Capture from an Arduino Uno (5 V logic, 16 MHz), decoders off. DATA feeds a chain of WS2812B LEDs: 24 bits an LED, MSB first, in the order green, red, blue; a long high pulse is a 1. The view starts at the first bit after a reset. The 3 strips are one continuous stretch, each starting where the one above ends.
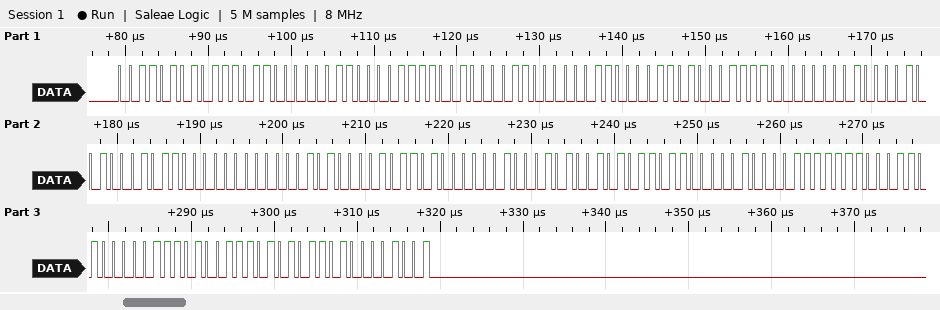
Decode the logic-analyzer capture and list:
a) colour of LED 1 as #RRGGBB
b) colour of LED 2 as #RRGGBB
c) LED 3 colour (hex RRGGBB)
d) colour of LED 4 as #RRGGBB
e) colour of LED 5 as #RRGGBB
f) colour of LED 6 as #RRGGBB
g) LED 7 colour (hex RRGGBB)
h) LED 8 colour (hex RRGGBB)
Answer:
#763506
#431E03
#1E0D01
#160900
#2D1402
#5B2904
#8D3F07
#AD4E09
